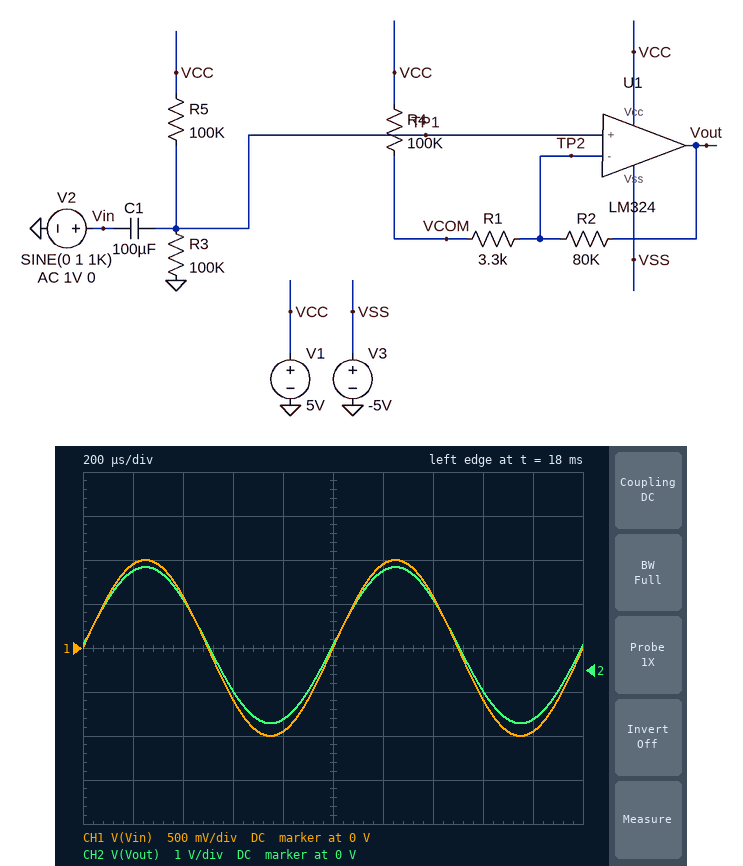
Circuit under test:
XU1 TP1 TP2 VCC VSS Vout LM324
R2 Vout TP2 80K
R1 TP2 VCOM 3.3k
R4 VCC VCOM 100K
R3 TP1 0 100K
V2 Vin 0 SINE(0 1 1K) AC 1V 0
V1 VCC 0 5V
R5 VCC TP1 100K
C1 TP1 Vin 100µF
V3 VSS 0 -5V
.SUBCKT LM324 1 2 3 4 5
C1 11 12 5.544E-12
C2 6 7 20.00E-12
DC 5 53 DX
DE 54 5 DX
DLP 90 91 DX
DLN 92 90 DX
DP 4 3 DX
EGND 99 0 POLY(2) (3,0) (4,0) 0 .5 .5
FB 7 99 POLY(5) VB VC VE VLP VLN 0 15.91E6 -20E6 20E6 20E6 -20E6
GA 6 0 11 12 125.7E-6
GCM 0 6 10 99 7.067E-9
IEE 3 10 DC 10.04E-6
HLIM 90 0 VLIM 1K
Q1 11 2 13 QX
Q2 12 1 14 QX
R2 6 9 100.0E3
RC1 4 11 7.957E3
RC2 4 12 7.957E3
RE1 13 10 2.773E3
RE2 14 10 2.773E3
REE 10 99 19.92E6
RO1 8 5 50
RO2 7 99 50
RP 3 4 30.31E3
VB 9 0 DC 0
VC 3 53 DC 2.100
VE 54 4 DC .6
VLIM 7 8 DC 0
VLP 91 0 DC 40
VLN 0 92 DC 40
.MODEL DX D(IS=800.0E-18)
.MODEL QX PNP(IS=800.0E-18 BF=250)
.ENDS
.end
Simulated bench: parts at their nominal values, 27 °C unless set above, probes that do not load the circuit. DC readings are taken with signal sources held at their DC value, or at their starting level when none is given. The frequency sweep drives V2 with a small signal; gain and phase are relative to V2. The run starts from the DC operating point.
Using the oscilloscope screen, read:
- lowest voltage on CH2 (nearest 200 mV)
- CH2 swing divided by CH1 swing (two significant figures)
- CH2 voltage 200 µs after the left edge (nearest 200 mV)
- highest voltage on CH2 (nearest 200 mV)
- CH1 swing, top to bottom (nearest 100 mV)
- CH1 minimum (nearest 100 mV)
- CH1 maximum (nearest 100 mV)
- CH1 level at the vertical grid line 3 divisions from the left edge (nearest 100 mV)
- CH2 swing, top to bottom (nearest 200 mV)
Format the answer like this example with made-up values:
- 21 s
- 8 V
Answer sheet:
- -1.2 V
- 1.8
- 2.2 V
- 2.4 V
- 2.0 V
- -1.0 V
- 1.0 V
- -600 mV
- 3.6 V
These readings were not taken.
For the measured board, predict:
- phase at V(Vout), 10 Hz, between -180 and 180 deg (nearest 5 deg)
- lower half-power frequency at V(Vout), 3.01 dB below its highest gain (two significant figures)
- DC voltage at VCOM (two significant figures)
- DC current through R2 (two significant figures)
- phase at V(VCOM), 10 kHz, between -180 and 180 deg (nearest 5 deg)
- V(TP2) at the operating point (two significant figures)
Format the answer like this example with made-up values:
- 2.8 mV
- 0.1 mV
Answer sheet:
- 0 deg
- 32 mHz
- 2.6 V
- 24 µA
- 0 deg
- 2.5 V
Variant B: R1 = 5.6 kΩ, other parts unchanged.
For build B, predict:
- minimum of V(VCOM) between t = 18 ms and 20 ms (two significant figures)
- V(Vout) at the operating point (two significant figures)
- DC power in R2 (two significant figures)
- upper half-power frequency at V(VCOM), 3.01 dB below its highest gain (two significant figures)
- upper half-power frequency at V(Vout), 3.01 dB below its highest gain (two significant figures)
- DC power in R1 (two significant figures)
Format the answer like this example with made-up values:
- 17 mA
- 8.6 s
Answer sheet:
- 1.7 V
- 610 mV
- 45 µW
- 740 kHz
- 750 kHz
- 3.1 µW
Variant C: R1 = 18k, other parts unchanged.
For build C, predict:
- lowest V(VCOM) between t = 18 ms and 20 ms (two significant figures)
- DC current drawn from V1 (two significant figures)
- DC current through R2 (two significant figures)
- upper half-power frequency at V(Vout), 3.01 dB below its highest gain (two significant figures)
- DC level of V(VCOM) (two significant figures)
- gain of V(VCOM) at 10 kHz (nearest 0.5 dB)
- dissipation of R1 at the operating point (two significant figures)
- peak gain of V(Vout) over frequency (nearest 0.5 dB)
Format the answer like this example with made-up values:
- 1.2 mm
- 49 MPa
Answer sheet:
- 2.0 V
- 390 µA
- 21 µA
- 790 kHz
- 2.9 V
- -1.5 dB
- 8.1 µW
- 4.5 dB
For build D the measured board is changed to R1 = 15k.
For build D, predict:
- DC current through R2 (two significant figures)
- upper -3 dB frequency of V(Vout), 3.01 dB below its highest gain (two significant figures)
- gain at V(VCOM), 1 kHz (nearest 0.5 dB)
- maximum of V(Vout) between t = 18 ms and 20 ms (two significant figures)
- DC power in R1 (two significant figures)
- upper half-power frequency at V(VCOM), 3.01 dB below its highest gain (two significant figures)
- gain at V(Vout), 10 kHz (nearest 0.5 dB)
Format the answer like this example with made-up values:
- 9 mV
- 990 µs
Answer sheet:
- 22 µA
- 780 kHz
- -1.0 dB
- 2.5 V
- 7.1 µW
- 770 kHz
- 4.5 dB
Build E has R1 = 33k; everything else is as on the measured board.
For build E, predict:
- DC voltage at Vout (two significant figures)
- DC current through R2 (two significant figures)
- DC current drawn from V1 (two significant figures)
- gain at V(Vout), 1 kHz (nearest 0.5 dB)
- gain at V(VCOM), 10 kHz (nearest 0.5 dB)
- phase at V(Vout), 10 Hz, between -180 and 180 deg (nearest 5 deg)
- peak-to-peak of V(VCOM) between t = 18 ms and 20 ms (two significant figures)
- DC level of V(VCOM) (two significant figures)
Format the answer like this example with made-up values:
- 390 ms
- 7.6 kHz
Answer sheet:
- 1.0 V
- 19 µA
- 380 µA
- 4.0 dB
- -2.5 dB
- 0 deg
- 1.5 V
- 3.1 V
